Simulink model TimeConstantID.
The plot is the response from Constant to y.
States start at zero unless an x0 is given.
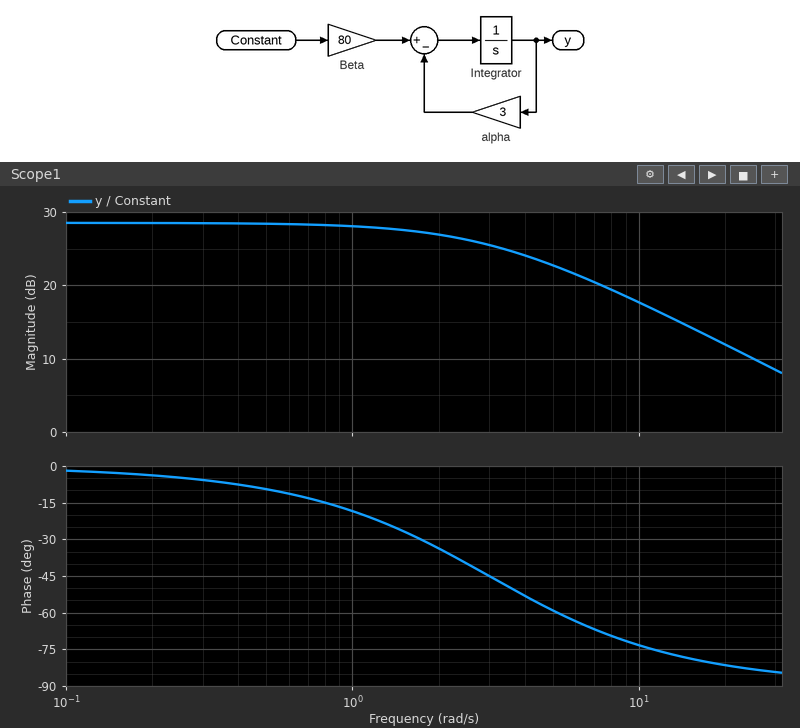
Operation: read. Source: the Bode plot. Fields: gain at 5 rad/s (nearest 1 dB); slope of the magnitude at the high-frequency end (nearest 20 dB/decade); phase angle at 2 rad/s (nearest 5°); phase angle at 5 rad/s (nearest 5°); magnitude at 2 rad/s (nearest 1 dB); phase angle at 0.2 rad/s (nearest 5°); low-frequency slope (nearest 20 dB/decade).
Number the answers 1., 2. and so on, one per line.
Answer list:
1. 23 dB
2. -20 dB/decade
3. -35°
4. -60°
5. 27 dB
6. -5°
7. 0 dB/decade
